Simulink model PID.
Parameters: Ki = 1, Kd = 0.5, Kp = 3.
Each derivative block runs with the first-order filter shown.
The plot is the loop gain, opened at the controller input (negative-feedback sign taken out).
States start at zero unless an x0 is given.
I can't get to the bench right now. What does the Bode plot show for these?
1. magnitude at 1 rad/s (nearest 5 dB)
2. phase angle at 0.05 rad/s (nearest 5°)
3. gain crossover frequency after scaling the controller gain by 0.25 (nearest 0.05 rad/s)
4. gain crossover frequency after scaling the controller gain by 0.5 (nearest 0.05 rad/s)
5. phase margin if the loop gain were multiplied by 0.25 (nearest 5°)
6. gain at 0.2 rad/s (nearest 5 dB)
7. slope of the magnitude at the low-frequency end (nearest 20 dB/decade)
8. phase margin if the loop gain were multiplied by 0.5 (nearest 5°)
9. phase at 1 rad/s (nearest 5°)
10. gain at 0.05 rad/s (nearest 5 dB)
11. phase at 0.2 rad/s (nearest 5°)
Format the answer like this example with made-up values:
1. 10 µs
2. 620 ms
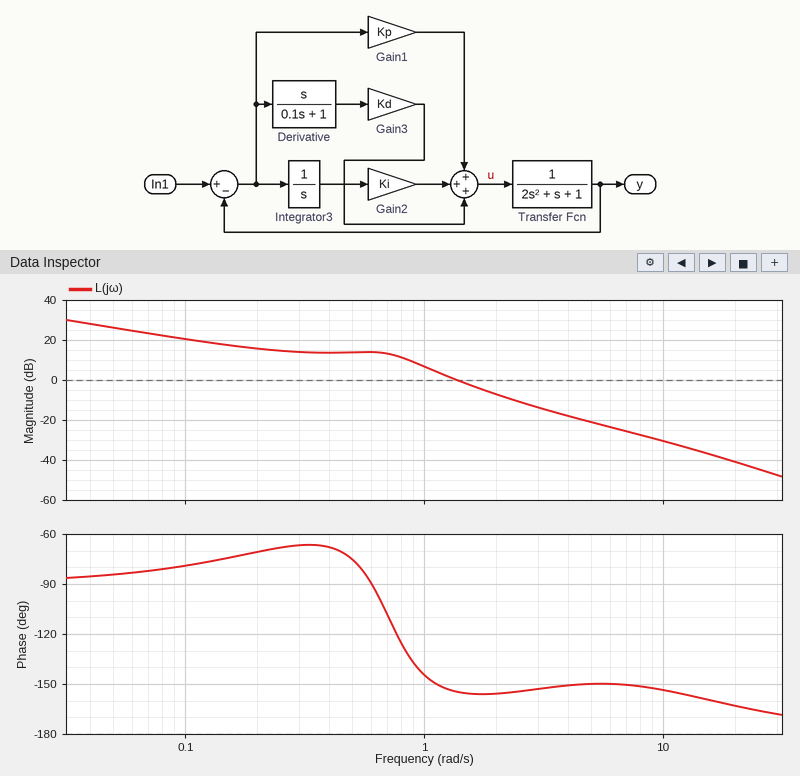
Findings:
1. 5 dB
2. -85°
3. 0.75 rad/s
4. 1.05 rad/s
5. 60°
6. 15 dB
7. -20 dB/decade
8. 35°
9. -145°
10. 25 dB
11. -70°
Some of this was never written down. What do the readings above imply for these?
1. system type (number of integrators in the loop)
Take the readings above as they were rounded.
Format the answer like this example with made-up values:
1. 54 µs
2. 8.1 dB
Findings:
1. 1
